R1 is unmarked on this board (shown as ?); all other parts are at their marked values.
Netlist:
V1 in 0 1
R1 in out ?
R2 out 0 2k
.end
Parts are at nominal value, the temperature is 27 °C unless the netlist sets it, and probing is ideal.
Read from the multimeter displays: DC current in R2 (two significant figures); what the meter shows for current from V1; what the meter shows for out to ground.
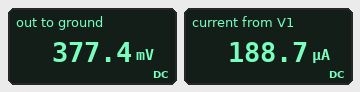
190 µA
188.7 µA
377.4 mV
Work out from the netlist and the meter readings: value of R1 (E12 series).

3.3 kΩ
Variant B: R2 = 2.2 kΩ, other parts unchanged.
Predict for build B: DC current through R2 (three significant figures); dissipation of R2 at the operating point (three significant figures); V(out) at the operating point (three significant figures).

182 µA
72.7 µW
400 mV
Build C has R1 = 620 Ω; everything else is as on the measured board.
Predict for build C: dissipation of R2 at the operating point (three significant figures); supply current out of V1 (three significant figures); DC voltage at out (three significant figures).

291 µW
382 µA
763 mV
